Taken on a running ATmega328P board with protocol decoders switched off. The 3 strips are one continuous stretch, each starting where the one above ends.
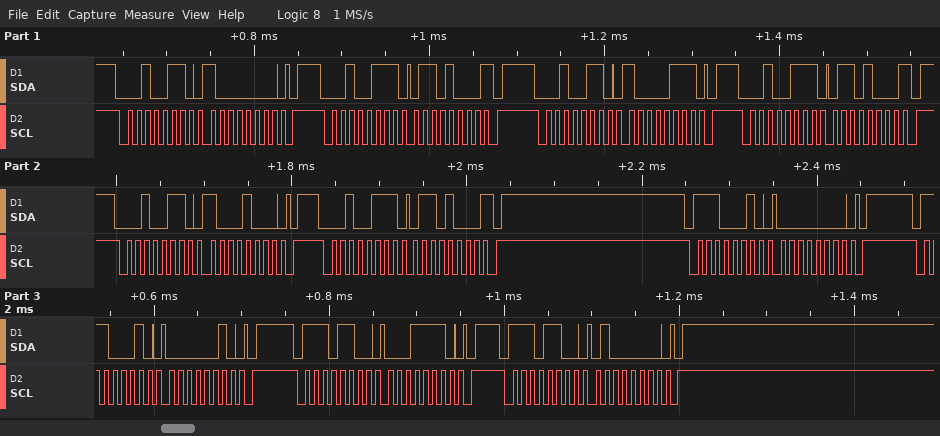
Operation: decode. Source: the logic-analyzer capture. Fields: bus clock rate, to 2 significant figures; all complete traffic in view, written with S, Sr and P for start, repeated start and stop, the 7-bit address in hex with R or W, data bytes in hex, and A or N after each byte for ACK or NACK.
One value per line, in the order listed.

100 kHz
S 13W A 80 A P S 13R A 68 N P S 13W A 87 A P S 13R A 68 N P S 13W A 88 A P S 13R A 68 N P S 71W A 00 A P S 71W A 02 A P S 76W A 1E A P S 76W A 40 A P
